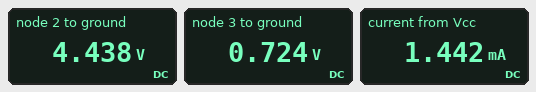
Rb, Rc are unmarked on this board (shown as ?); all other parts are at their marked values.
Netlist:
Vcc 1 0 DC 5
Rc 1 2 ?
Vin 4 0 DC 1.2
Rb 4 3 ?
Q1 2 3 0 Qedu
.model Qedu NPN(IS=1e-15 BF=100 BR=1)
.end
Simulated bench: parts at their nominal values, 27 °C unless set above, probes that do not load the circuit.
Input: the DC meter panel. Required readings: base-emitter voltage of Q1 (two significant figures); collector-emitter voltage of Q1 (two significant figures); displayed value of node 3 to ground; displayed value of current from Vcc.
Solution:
720 mV
4.4 V
0.724 V
1.442 mA
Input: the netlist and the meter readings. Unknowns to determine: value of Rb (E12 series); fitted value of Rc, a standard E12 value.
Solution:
33 kΩ
390 Ω
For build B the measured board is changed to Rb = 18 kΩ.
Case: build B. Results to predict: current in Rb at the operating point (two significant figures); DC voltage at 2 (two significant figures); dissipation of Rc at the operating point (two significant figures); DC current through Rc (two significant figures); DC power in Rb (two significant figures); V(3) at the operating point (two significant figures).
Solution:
26 µA
4.0 V
2.6 mW
2.6 mA
12 µW
740 mV
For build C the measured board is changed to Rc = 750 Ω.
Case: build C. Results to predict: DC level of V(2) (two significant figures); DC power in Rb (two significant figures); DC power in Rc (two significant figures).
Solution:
3.9 V
6.9 µW
1.6 mW
